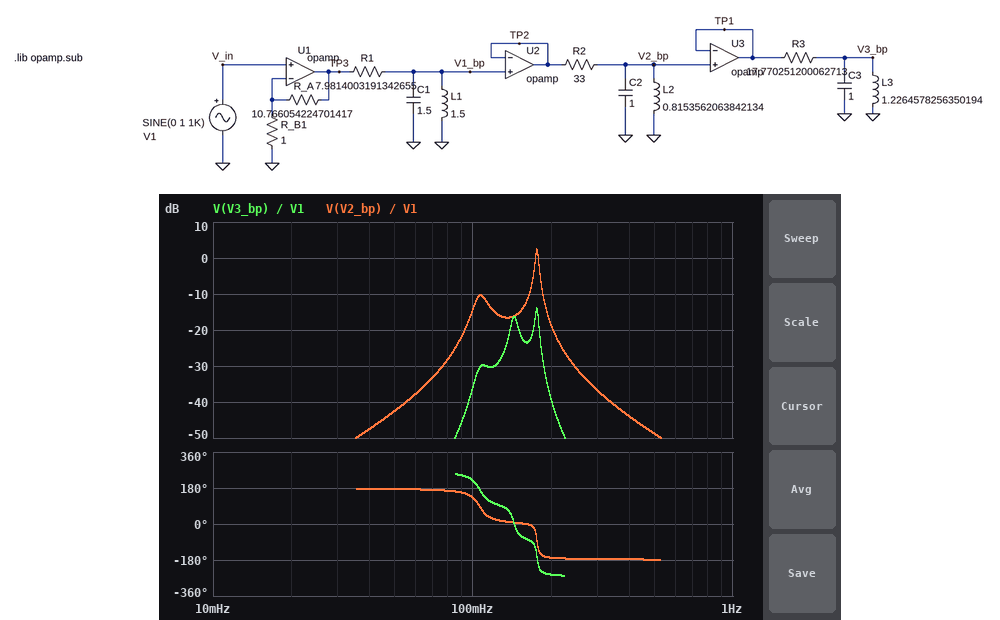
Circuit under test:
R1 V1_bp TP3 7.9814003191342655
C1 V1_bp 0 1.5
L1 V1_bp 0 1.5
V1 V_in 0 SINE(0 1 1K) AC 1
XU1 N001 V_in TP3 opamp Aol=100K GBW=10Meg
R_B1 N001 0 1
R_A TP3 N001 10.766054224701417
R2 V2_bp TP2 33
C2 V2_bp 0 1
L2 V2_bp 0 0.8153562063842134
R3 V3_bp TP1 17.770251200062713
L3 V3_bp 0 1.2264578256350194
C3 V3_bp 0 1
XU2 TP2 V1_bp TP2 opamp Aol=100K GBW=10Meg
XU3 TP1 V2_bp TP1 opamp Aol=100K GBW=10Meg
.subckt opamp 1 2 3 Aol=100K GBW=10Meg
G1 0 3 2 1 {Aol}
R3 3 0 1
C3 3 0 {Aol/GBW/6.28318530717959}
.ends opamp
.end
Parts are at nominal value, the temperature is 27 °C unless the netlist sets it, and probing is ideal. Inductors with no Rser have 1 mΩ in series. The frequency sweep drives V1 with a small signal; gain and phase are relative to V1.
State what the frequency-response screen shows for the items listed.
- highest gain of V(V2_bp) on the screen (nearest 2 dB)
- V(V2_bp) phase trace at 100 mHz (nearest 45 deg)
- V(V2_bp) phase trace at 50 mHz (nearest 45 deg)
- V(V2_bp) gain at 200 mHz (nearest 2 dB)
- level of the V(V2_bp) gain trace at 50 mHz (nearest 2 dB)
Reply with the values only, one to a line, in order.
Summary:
2 dB
135 deg
180 deg
-18 dB
-42 dB
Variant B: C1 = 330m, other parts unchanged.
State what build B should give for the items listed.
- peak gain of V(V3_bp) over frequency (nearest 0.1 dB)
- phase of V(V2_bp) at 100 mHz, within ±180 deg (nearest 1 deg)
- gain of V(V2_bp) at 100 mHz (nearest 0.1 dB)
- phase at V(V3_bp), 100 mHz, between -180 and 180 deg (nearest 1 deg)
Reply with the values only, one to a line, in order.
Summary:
-2.0 dB
170 deg
-28.2 dB
-105 deg
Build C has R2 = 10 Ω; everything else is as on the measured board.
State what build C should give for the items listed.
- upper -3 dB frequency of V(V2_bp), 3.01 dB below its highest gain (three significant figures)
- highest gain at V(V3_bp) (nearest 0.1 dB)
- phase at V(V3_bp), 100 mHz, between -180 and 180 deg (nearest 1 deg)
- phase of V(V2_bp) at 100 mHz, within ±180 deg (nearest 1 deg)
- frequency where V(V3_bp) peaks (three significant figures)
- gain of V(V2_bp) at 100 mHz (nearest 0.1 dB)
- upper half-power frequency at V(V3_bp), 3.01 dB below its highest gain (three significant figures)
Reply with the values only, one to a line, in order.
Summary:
183 mHz
-6.1 dB
-146 deg
129 deg
144 mHz
-3.9 dB
149 mHz
